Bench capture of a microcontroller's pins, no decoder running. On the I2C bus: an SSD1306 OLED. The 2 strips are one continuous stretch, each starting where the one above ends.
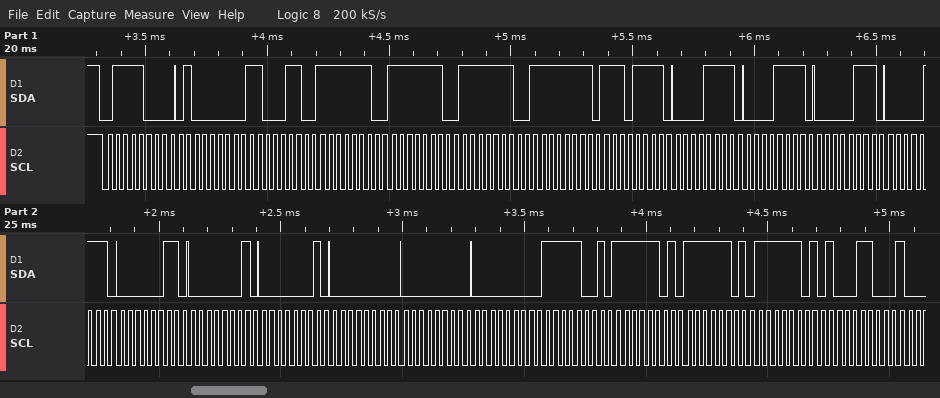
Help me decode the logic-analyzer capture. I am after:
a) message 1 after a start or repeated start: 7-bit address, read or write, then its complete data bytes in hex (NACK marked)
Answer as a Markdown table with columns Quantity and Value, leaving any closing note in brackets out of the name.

| Quantity | Value |
|---|---|
| message 1 after a start or repeated start: 7-bit address, read or write, then its complete data bytes in hex | 0x3C write: 40 C6 FE FE FE FF EF 0F 0F 07 07 03 01 01 00 00 00 F9 FD FD FD 8C |
